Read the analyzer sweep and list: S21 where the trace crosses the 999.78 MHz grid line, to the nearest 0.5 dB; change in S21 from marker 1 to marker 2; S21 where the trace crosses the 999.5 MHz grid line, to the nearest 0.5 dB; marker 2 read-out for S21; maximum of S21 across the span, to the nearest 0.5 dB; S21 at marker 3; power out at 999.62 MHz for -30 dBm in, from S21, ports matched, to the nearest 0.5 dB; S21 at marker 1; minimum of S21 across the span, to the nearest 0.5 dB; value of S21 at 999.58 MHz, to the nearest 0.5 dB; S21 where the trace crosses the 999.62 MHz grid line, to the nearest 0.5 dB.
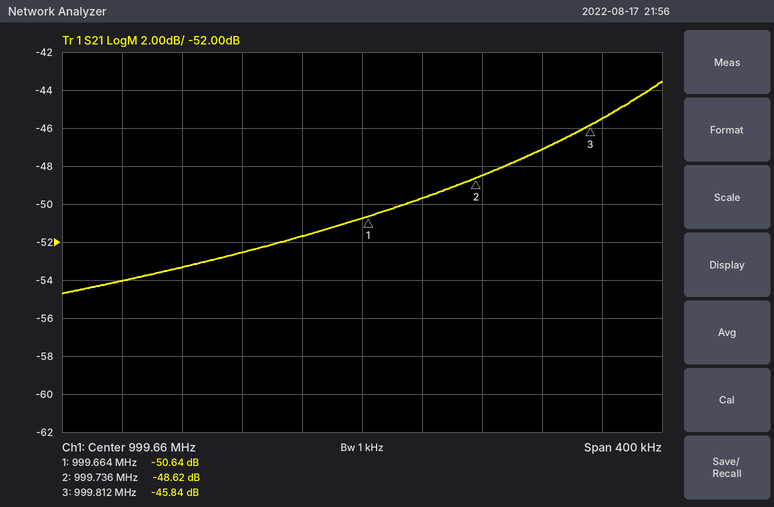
-47.0 dB
2.02 dB
-54.0 dB
-48.62 dB
-43.5 dB
-45.84 dB
-81.5 dBm
-50.64 dB
-54.5 dB
-52.5 dB
-51.5 dB
